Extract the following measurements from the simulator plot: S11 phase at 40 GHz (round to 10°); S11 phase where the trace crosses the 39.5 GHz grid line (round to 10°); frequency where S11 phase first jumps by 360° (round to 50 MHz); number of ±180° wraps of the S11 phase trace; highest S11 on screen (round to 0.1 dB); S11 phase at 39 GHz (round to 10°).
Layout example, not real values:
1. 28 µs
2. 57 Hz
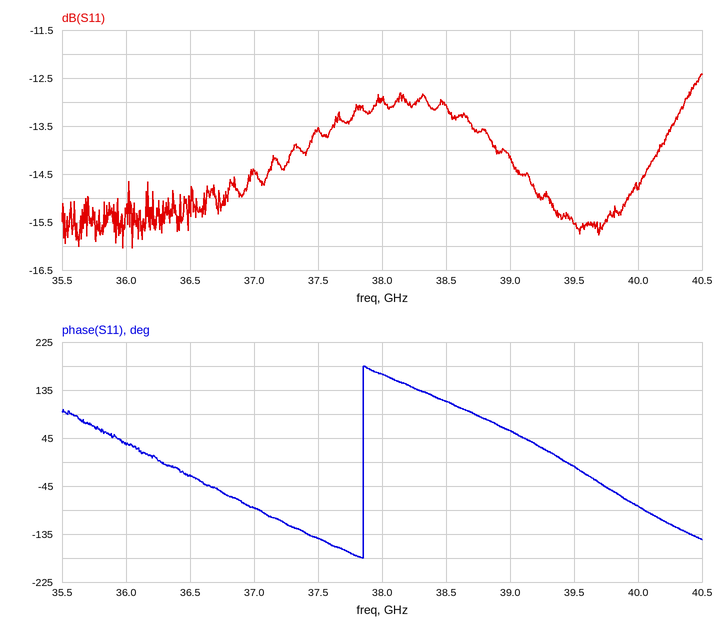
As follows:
1. -80°
2. -10°
3. 37.85 GHz
4. 1
5. -12.4 dB
6. 60°
